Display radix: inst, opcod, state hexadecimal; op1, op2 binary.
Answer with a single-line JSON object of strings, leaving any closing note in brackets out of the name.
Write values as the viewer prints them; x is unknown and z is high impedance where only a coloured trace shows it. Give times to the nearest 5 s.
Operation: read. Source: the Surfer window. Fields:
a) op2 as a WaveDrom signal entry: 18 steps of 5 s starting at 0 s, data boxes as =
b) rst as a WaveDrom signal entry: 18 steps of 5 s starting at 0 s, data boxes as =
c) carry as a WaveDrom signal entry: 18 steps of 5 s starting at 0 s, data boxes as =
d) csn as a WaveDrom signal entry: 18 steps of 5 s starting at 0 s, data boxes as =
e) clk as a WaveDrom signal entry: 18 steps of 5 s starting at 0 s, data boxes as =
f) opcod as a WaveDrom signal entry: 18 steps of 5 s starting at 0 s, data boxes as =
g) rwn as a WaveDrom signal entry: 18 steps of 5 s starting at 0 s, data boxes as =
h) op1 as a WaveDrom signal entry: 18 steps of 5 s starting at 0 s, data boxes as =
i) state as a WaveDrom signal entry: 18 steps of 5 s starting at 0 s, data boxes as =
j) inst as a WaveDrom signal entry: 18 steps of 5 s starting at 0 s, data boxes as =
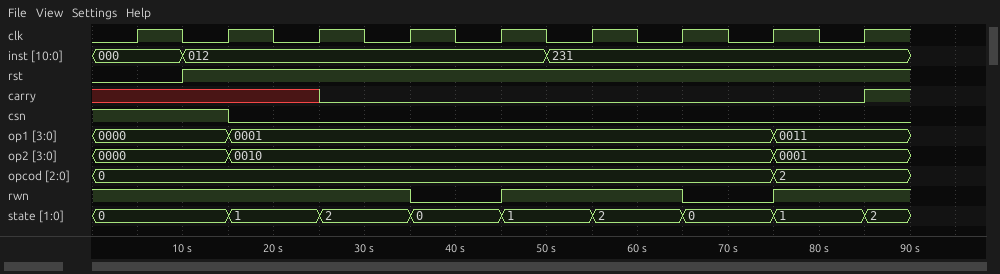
{"op2 as a WaveDrom signal entry: 18 steps of 5 s starting at 0 s, data boxes as =": "{name: 'op2', wave: '=..=...........=..', data: '0000 0010 0001'}", "rst as a WaveDrom signal entry: 18 steps of 5 s starting at 0 s, data boxes as =": "{name: 'rst', wave: '0.1...............'}", "carry as a WaveDrom signal entry: 18 steps of 5 s starting at 0 s, data boxes as =": "{name: 'carry', wave: 'x....0...........1'}", "csn as a WaveDrom signal entry: 18 steps of 5 s starting at 0 s, data boxes as =": "{name: 'csn', wave: '1..0..............'}", "clk as a WaveDrom signal entry: 18 steps of 5 s starting at 0 s, data boxes as =": "{name: 'clk', wave: '010101010101010101'}", "opcod as a WaveDrom signal entry: 18 steps of 5 s starting at 0 s, data boxes as =": "{name: 'opcod', wave: '=..............=..', data: '0 2'}", "rwn as a WaveDrom signal entry: 18 steps of 5 s starting at 0 s, data boxes as =": "{name: 'rwn', wave: '1......0.1...0.1..'}", "op1 as a WaveDrom signal entry: 18 steps of 5 s starting at 0 s, data boxes as =": "{name: 'op1', wave: '=..=...........=..', data: '0000 0001 0011'}", "state as a WaveDrom signal entry: 18 steps of 5 s starting at 0 s, data boxes as =": "{name: 'state', wave: '=..=.=.=.=.=.=.=.=', data: '0 1 2 0 1 2 0 1 2'}", "inst as a WaveDrom signal entry: 18 steps of 5 s starting at 0 s, data boxes as =": "{name: 'inst', wave: '=.=.......=.......', data: '000 012 231'}"}
